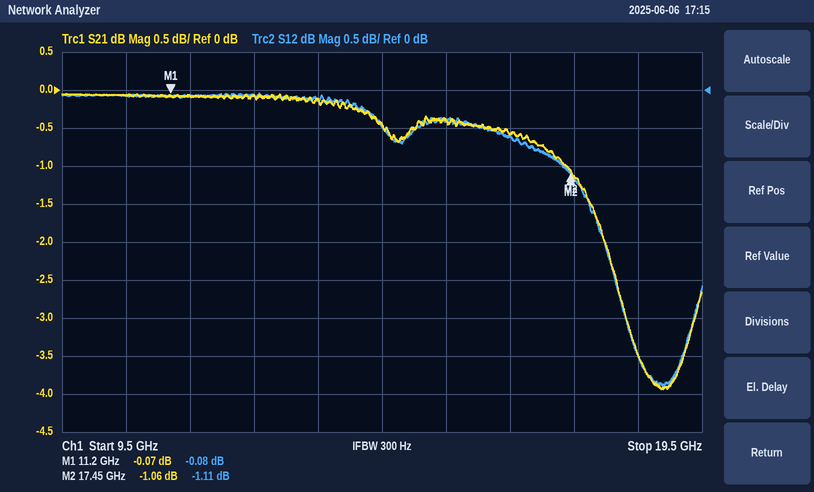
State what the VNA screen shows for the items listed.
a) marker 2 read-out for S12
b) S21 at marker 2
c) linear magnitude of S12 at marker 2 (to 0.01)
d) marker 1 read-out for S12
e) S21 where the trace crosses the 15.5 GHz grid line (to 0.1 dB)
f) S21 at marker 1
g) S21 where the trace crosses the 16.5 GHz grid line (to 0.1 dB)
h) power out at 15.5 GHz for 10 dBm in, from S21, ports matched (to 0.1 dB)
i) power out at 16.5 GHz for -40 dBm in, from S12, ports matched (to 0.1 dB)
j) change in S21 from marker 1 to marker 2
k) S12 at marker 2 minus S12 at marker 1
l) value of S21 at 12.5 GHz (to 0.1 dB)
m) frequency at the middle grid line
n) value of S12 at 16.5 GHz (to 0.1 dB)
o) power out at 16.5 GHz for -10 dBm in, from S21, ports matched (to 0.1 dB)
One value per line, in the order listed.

-1.11 dB
-1.06 dB
0.88
-0.08 dB
-0.4 dB
-0.07 dB
-0.6 dB
9.6 dBm
-40.6 dBm
-0.99 dB
-1.03 dB
-0.1 dB
14.5 GHz
-0.6 dB
-10.6 dBm
